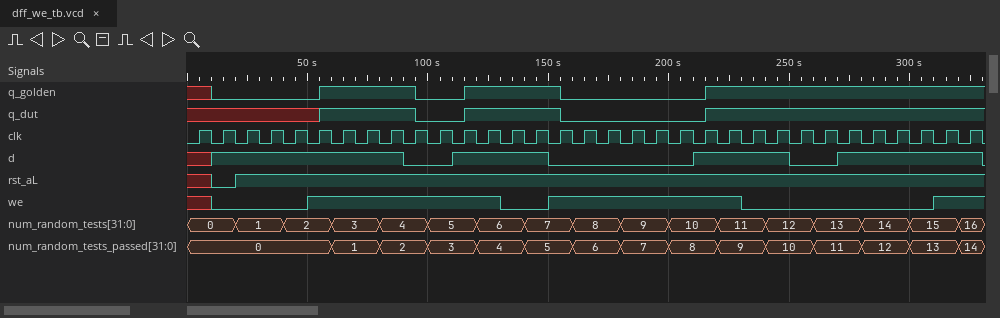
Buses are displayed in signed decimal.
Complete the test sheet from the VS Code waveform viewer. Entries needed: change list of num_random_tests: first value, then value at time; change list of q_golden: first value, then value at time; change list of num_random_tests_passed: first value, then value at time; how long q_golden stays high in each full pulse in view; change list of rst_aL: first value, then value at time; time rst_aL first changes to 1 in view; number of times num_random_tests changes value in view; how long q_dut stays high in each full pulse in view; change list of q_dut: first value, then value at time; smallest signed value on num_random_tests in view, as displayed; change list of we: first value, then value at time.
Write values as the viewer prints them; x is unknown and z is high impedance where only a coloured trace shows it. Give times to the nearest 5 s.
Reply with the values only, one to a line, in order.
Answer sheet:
0, 1 at 20 s, 2 at 40 s, 3 at 60 s, 4 at 80 s, 5 at 100 s, 6 at 120 s, 7 at 140 s, 8 at 160 s, 9 at 180 s, 10 at 200 s, 11 at 220 s, 12 at 240 s, 13 at 260 s, 14 at 280 s, 15 at 300 s, 16 at 320 s
x, 0 at 10 s, 1 at 55 s, 0 at 95 s, 1 at 115 s, 0 at 155 s, 1 at 215 s
0, 1 at 60 s, 2 at 80 s, 3 at 100 s, 4 at 120 s, 5 at 140 s, 6 at 160 s, 7 at 180 s, 8 at 200 s, 9 at 220 s, 10 at 240 s, 11 at 260 s, 12 at 280 s, 13 at 300 s, 14 at 320 s
40 s, 40 s
x, 0 at 10 s, 1 at 20 s
20 s
16
40 s
x, 1 at 55 s, 0 at 95 s, 1 at 115 s, 0 at 155 s, 1 at 215 s
0
x, 0 at 10 s, 1 at 50 s, 0 at 130 s, 1 at 150 s, 0 at 230 s, 1 at 310 s
